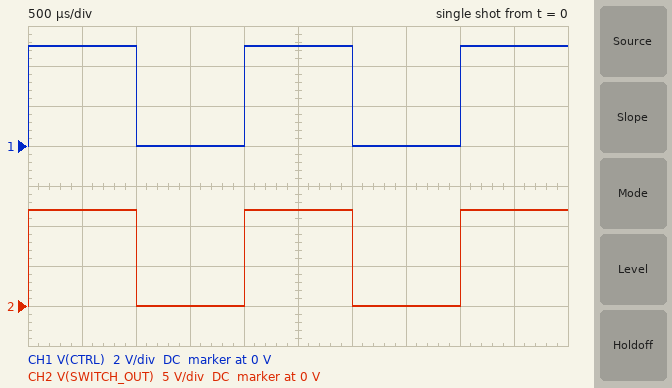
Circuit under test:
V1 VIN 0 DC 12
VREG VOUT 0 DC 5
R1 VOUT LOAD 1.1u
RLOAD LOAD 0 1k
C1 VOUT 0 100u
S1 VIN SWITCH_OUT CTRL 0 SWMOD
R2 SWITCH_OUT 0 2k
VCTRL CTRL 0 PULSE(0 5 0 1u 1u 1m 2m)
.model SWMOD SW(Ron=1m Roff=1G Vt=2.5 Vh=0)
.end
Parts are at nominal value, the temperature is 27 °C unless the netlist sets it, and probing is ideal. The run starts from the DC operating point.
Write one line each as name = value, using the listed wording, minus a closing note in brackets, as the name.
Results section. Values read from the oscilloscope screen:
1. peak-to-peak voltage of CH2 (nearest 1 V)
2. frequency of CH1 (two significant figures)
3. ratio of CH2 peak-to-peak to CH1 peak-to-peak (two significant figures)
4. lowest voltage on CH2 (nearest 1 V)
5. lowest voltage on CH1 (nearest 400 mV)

peak-to-peak voltage of CH2 = 12 V
frequency of CH1 = 500 Hz
ratio of CH2 peak-to-peak to CH1 peak-to-peak = 2.4
lowest voltage on CH2 = 0 V
lowest voltage on CH1 = 0 V
